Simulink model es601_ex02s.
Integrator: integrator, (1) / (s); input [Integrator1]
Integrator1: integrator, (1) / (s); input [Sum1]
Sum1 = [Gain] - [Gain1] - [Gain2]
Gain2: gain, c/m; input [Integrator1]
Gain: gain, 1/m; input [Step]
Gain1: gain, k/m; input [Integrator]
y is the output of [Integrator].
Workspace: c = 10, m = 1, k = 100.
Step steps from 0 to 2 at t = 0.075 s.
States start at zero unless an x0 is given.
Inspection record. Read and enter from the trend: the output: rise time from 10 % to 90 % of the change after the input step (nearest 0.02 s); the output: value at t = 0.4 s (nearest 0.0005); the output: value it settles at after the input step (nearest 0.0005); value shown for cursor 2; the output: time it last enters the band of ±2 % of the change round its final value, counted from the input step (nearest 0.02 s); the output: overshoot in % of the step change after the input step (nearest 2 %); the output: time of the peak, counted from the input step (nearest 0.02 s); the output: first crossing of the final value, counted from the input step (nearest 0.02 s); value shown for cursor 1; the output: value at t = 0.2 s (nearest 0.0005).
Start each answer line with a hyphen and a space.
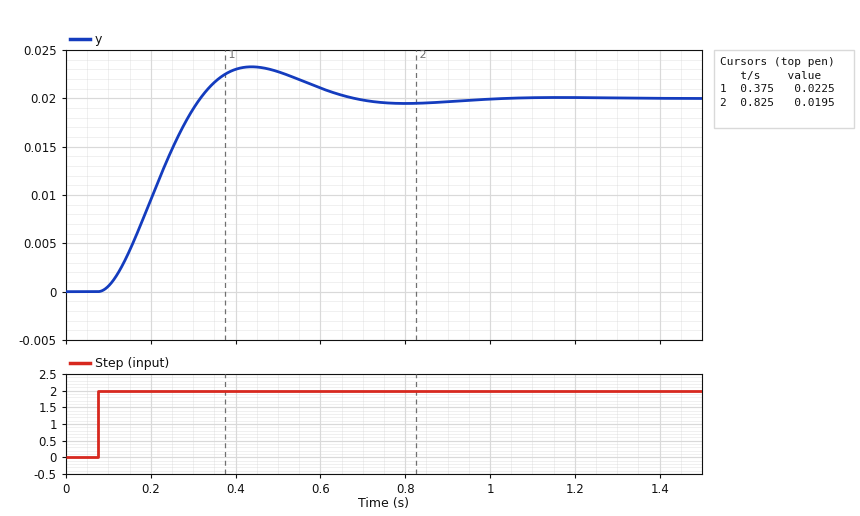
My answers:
- 0.16 s
- 0.0230
- 0.0200
- 0.0195
- 0.80 s
- 16 %
- 0.36 s
- 0.24 s
- 0.0225
- 0.0095
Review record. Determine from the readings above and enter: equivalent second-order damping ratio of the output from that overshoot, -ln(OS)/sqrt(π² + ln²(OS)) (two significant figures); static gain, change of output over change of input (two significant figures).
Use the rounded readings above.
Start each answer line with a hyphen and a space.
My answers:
- 0.50
- 0.010
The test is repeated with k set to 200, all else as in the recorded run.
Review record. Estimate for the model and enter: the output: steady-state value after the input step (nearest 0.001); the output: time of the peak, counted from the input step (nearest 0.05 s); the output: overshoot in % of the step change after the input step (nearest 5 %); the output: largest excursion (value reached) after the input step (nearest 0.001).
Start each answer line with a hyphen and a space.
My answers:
- 0.010
- 0.25 s
- 30 %
- 0.013
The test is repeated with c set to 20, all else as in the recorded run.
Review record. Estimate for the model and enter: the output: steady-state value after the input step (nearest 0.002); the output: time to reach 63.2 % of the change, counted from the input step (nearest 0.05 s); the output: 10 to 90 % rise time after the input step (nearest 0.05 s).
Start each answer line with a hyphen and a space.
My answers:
- 0.020
- 0.20 s
- 0.35 s
